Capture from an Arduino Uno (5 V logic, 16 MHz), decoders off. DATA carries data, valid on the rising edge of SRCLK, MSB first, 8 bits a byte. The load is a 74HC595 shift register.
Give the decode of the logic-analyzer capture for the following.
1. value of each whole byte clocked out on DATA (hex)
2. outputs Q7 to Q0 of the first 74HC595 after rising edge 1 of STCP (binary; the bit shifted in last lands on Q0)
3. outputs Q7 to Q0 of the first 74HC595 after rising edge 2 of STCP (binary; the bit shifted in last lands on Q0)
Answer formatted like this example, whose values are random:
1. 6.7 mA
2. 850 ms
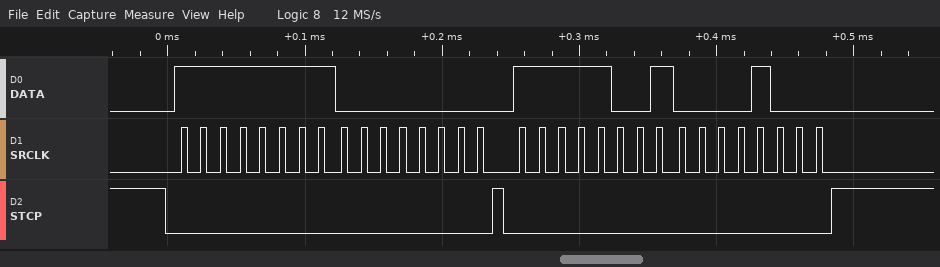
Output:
1. FF 00 F9 08
2. 00000000
3. 00001000
